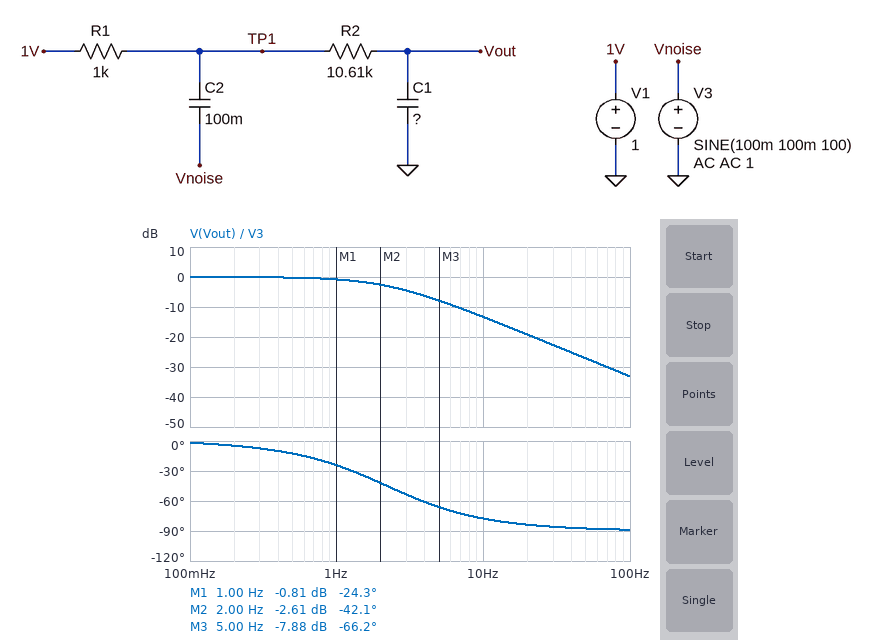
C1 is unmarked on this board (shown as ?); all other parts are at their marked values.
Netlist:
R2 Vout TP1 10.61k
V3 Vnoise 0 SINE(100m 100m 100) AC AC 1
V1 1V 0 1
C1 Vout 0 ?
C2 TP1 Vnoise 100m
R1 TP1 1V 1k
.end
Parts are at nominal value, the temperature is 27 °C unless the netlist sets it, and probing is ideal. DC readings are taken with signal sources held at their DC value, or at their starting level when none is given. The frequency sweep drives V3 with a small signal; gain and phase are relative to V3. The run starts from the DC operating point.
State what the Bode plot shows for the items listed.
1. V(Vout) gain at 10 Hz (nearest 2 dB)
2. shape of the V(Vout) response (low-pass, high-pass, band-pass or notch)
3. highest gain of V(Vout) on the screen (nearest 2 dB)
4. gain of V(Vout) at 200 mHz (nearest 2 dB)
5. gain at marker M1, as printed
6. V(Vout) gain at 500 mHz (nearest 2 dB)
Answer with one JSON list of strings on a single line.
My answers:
["-14 dB", "low-pass", "0 dB", "0 dB", "-0.81 dB", "0 dB"]
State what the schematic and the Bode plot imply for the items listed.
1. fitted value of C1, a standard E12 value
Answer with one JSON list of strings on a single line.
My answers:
["6.8 µF"]
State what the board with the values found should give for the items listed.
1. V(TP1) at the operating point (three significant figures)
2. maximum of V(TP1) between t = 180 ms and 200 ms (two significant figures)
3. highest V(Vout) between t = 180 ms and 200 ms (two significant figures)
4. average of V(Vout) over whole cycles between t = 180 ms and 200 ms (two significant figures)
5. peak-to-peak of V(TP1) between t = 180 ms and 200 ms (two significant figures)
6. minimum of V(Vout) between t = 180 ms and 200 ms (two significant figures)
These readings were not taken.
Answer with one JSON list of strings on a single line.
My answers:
["1.00 V", "1.1 V", "1.0 V", "1.0 V", "200 mV", "1.0 V"]
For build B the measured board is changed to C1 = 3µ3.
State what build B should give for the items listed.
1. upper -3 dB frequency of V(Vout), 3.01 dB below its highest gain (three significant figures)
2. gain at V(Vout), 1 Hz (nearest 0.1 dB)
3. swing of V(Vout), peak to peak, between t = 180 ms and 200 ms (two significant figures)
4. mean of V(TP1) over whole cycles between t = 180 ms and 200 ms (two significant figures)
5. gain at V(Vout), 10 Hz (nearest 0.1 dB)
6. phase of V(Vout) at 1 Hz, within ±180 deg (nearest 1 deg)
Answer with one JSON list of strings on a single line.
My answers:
["4.55 Hz", "-0.2 dB", "9.1 mV", "1.0 V", "-7.7 dB", "-12 deg"]
